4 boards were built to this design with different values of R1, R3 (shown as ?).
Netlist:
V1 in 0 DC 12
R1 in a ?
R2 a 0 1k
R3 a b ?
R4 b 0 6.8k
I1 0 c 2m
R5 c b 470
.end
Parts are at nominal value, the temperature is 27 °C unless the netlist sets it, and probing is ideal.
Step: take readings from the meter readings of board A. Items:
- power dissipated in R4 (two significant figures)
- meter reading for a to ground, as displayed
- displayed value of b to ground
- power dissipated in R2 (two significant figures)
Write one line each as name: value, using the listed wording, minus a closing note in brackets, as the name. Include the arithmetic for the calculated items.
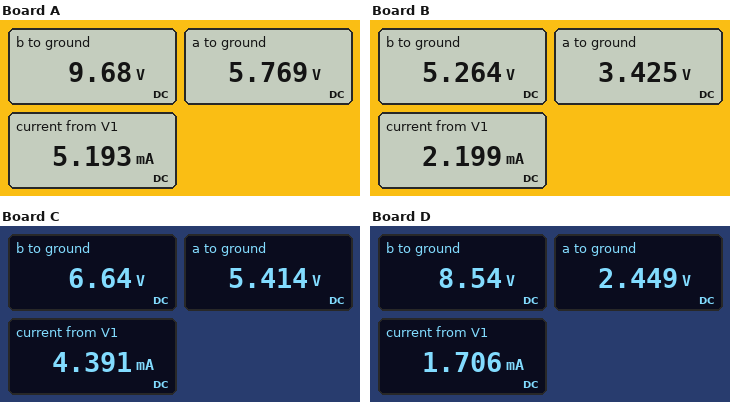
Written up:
power dissipated in R4: (9.68 V)^2 / 6.8 kΩ = 14 mW
meter reading for a to ground, as displayed: 5.769 V
displayed value of b to ground: 9.68 V
power dissipated in R2: (5.769 V)^2 / 1 kΩ = 33 mW
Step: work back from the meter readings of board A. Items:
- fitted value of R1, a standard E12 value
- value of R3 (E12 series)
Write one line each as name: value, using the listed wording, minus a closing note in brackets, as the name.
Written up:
fitted value of R1, a standard E12 value: 1.2 kΩ
value of R3: 6.8 kΩ
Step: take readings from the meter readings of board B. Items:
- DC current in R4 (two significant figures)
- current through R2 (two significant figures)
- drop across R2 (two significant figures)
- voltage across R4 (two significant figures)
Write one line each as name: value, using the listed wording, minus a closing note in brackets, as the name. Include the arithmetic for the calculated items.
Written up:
DC current in R4: (5.264 V) / 6.8 kΩ = 770 µA
current through R2: (3.425 V) / 1 kΩ = 3.4 mA
drop across R2: 3.425 V = 3.4 V
voltage across R4: 5.264 V = 5.3 V
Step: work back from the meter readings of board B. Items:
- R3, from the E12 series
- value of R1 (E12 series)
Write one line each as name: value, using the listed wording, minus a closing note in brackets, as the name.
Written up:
R3, from the E12 series: 1.5 kΩ
value of R1: 3.9 kΩ
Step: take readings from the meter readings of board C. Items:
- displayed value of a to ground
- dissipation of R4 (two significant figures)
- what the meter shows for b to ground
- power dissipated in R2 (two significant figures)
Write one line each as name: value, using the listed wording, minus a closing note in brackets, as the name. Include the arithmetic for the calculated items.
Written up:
displayed value of a to ground: 5.414 V
dissipation of R4: (6.64 V)^2 / 6.8 kΩ = 6.5 mW
what the meter shows for b to ground: 6.64 V
power dissipated in R2: (5.414 V)^2 / 1 kΩ = 29 mW
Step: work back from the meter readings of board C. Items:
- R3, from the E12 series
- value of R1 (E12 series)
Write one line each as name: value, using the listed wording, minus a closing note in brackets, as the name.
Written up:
R3, from the E12 series: 1.2 kΩ
value of R1: 1.5 kΩ
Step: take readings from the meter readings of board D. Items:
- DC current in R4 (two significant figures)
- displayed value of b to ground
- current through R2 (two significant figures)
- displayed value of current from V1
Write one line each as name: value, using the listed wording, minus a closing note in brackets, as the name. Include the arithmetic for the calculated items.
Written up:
DC current in R4: (8.54 V) / 6.8 kΩ = 1.3 mA
displayed value of b to ground: 8.54 V
current through R2: (2.449 V) / 1 kΩ = 2.4 mA
displayed value of current from V1: 1.706 mA
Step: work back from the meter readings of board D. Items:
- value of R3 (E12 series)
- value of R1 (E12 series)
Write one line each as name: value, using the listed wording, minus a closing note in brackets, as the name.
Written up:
value of R3: 8.2 kΩ
value of R1: 5.6 kΩ
